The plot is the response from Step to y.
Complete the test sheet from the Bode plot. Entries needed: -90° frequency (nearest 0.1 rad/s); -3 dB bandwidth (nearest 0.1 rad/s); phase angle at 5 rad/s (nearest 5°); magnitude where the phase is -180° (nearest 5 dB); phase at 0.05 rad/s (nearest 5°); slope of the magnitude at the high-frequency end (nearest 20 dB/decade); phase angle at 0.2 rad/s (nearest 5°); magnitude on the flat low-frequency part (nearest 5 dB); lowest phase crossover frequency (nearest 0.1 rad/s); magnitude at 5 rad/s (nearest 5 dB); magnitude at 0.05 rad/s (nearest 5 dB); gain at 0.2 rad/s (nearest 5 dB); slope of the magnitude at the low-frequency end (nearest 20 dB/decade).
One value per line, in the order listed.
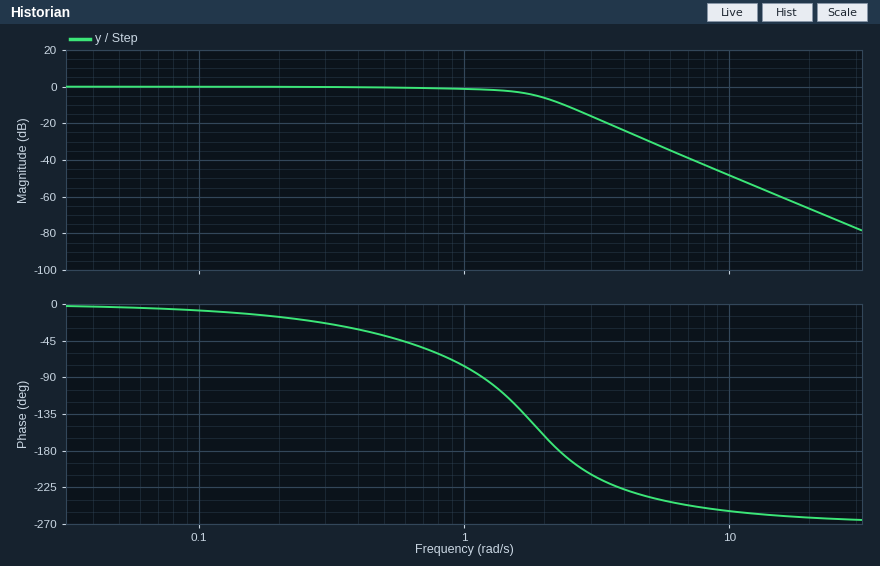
1.2 rad/s
1.6 rad/s
-235°
-10 dB
-5°
-60 dB/decade
-15°
0 dB
2.3 rad/s
-30 dB
0 dB
0 dB
0 dB/decade
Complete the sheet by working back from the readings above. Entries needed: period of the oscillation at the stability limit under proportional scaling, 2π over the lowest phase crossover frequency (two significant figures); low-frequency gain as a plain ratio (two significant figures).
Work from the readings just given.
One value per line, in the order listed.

2.7 s
1.0
